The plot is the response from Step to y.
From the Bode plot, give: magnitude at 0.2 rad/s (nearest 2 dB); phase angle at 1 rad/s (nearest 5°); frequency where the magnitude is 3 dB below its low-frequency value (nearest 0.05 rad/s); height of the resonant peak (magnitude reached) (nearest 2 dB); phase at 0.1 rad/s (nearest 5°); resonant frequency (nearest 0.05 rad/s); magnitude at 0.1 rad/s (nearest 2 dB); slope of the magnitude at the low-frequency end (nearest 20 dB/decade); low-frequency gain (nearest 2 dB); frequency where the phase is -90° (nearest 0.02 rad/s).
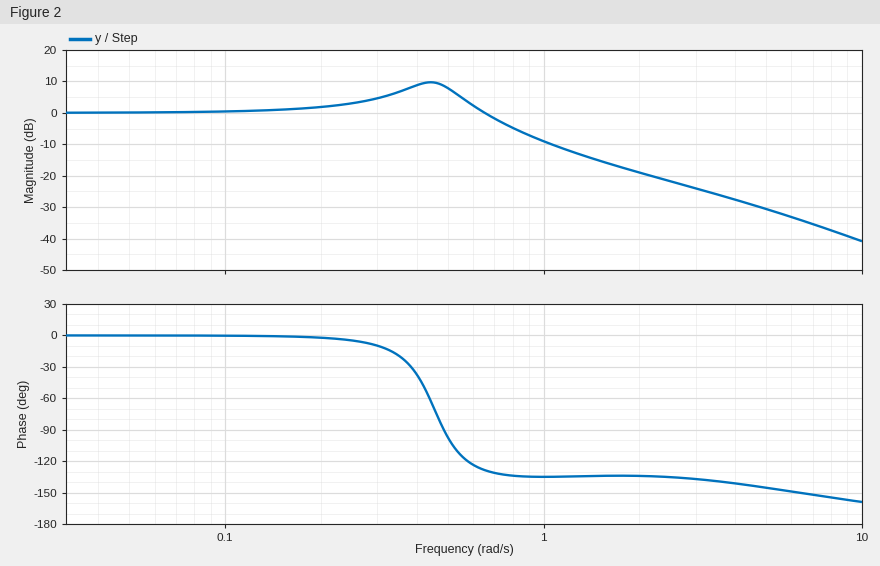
2 dB
-135°
0.75 rad/s
10 dB
0°
0.45 rad/s
0 dB
0 dB/decade
0 dB
0.48 rad/s
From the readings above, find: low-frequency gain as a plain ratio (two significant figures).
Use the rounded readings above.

1.0
